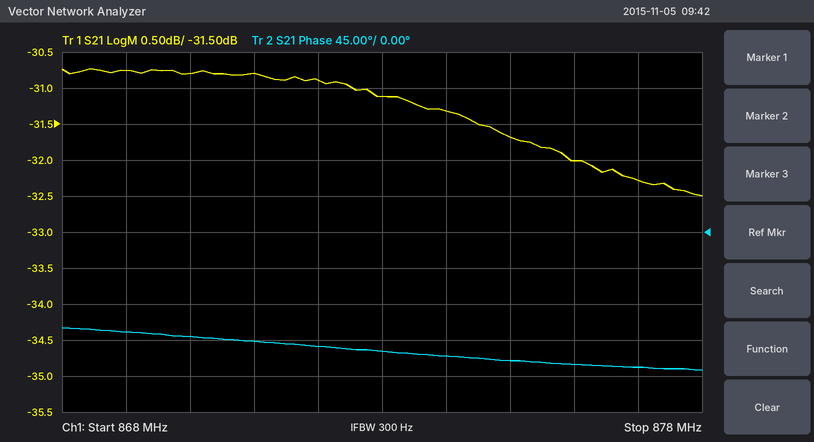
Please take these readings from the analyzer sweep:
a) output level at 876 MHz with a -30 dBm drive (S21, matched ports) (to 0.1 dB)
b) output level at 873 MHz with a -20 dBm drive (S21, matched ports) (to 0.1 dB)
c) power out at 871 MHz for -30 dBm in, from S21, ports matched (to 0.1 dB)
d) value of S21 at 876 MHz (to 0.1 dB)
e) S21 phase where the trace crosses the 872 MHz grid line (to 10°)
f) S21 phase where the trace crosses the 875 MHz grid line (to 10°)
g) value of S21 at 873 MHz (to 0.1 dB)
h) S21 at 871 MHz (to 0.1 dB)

-62.0 dBm
-51.1 dBm
-60.8 dBm
-32.0 dB
-140°
-160°
-31.1 dB
-30.8 dB
